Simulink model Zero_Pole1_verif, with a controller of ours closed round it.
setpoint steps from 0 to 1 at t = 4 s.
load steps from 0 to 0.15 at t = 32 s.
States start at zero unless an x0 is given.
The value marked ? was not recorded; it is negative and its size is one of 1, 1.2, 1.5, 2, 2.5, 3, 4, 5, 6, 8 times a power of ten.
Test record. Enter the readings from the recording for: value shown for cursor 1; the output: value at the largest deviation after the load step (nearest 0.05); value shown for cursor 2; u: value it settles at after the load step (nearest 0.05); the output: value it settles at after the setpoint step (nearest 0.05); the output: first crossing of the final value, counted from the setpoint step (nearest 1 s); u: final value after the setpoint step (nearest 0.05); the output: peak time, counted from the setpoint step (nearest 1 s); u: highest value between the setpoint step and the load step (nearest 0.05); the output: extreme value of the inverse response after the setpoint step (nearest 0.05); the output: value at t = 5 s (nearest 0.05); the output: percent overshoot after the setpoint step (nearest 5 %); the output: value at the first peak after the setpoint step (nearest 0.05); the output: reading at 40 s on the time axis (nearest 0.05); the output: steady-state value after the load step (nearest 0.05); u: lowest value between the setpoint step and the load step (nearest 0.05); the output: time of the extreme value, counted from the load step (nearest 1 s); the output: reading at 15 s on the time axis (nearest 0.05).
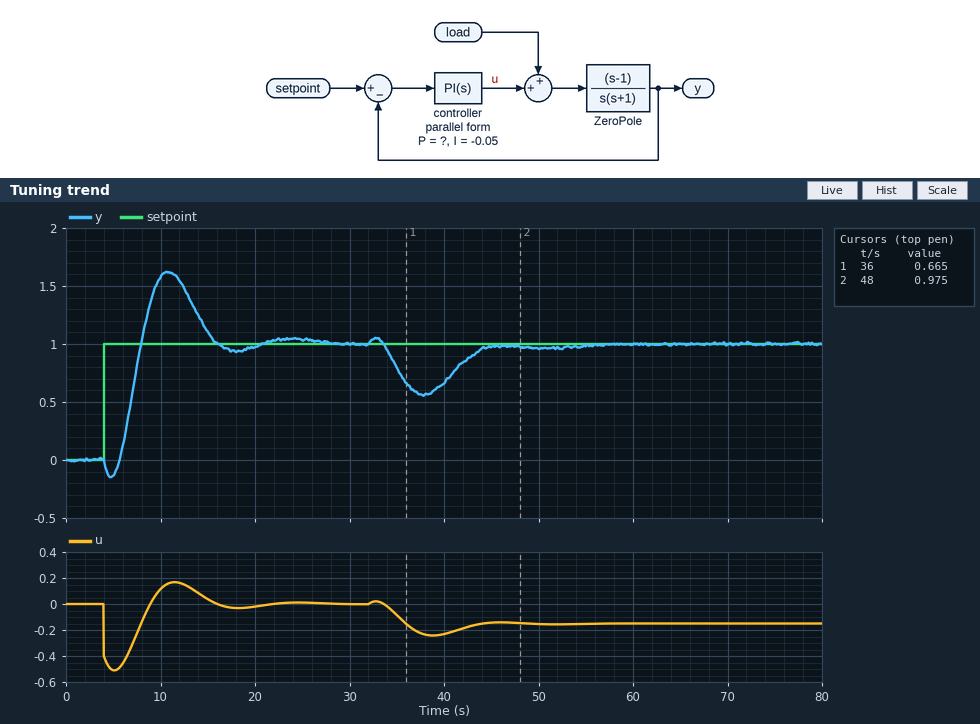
0.665
0.55
0.975
-0.15
1.00
4 s
0.00
7 s
0.15
-0.15
-0.15
60 %
1.60
0.65
1.00
-0.50
6 s
1.10
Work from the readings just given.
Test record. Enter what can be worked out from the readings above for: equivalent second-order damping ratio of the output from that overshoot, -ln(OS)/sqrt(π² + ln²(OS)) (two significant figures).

0.16
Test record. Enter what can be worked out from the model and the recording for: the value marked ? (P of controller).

-0.4
